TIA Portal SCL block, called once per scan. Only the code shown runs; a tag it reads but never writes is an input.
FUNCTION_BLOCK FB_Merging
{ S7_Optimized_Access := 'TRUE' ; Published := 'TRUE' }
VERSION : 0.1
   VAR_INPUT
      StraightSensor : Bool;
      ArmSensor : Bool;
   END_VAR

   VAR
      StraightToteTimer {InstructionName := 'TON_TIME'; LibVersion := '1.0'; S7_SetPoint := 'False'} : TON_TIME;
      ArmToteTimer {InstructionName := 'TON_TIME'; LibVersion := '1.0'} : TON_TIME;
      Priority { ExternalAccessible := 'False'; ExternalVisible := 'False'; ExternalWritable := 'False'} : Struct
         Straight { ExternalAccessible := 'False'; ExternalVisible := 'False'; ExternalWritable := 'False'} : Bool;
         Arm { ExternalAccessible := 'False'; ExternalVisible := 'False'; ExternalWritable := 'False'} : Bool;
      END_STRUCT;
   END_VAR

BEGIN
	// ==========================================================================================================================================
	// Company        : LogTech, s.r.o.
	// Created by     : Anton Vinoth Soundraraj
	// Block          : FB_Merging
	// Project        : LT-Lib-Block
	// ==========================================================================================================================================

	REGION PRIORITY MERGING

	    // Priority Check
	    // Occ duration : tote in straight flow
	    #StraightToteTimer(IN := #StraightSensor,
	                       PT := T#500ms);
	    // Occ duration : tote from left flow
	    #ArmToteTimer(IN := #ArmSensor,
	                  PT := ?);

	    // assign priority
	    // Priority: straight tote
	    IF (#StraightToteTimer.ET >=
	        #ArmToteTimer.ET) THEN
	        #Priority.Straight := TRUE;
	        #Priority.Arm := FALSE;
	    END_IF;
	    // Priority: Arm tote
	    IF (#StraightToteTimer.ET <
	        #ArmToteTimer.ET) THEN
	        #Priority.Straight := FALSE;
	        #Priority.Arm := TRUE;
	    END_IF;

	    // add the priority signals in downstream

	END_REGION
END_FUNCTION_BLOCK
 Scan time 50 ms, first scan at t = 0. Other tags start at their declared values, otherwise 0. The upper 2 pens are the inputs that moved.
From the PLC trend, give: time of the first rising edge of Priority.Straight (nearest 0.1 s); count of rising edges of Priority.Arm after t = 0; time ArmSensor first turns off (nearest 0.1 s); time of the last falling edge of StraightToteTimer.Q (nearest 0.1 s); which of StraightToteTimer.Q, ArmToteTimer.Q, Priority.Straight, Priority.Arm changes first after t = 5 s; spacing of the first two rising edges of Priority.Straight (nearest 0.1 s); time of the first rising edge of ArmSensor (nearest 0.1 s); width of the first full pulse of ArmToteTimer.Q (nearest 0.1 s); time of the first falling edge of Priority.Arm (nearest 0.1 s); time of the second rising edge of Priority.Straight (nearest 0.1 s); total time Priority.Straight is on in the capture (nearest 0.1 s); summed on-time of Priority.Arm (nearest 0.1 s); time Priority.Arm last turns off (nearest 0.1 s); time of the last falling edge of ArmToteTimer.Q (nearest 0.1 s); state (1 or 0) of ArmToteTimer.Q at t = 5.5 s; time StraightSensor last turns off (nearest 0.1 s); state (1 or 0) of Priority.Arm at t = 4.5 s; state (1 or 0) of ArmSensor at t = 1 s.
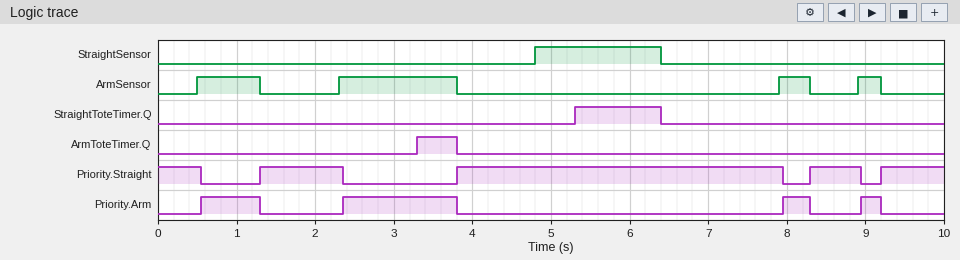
1.3 s
4
1.3 s
6.4 s
StraightToteTimer.Q
2.5 s
0.5 s
0.5 s
1.3 s
3.8 s
7.2 s
2.8 s
9.2 s
3.8 s
0
6.4 s
0
1
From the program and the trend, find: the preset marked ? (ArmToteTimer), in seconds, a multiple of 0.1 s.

1.0 s
